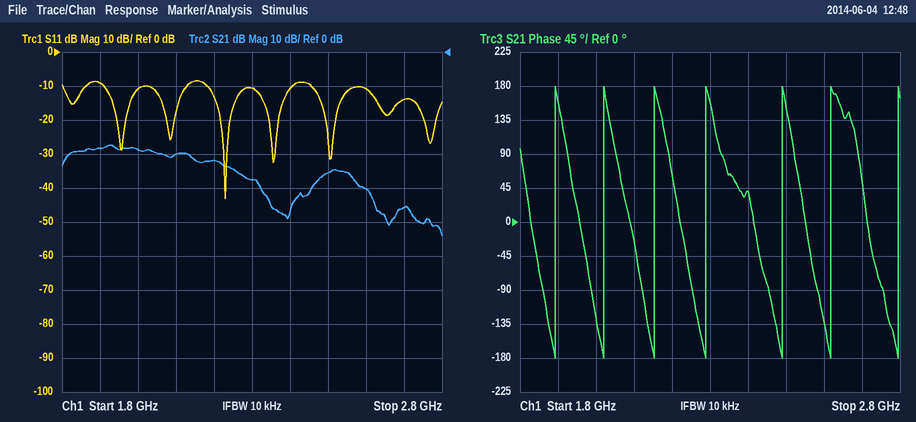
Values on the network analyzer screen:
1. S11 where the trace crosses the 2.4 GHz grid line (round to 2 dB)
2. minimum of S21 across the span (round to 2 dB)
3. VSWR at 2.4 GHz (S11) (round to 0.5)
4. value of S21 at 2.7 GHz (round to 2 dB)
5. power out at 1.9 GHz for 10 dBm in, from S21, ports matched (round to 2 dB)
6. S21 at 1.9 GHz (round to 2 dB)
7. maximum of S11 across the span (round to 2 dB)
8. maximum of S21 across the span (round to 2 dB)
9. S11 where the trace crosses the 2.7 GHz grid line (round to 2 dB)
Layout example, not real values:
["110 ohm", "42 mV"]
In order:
["-10 dB", "-54 dB", "2.0", "-46 dB", "-18 dBm", "-28 dB", "-8 dB", "-28 dB", "-14 dB"]
